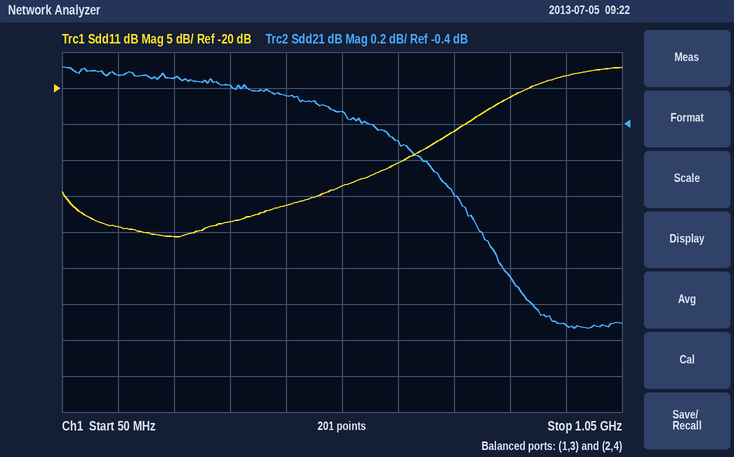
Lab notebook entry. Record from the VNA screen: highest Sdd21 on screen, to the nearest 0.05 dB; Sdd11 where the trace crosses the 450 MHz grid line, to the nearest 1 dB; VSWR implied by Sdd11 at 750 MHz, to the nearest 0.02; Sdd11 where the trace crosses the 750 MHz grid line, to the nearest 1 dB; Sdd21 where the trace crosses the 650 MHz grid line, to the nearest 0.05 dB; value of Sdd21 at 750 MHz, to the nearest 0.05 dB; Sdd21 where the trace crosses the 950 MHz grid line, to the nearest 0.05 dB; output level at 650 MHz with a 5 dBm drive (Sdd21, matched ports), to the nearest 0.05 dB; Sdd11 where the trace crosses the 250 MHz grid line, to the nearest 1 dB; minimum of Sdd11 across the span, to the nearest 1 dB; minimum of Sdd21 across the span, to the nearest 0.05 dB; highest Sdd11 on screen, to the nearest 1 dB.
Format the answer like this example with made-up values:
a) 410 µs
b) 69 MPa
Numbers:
a) -0.10 dB
b) -36 dB
c) 1.10
d) -26 dB
e) -0.50 dB
f) -0.80 dB
g) -1.50 dB
h) 4.50 dBm
i) -41 dB
j) -41 dB
k) -1.55 dB
l) -17 dB
